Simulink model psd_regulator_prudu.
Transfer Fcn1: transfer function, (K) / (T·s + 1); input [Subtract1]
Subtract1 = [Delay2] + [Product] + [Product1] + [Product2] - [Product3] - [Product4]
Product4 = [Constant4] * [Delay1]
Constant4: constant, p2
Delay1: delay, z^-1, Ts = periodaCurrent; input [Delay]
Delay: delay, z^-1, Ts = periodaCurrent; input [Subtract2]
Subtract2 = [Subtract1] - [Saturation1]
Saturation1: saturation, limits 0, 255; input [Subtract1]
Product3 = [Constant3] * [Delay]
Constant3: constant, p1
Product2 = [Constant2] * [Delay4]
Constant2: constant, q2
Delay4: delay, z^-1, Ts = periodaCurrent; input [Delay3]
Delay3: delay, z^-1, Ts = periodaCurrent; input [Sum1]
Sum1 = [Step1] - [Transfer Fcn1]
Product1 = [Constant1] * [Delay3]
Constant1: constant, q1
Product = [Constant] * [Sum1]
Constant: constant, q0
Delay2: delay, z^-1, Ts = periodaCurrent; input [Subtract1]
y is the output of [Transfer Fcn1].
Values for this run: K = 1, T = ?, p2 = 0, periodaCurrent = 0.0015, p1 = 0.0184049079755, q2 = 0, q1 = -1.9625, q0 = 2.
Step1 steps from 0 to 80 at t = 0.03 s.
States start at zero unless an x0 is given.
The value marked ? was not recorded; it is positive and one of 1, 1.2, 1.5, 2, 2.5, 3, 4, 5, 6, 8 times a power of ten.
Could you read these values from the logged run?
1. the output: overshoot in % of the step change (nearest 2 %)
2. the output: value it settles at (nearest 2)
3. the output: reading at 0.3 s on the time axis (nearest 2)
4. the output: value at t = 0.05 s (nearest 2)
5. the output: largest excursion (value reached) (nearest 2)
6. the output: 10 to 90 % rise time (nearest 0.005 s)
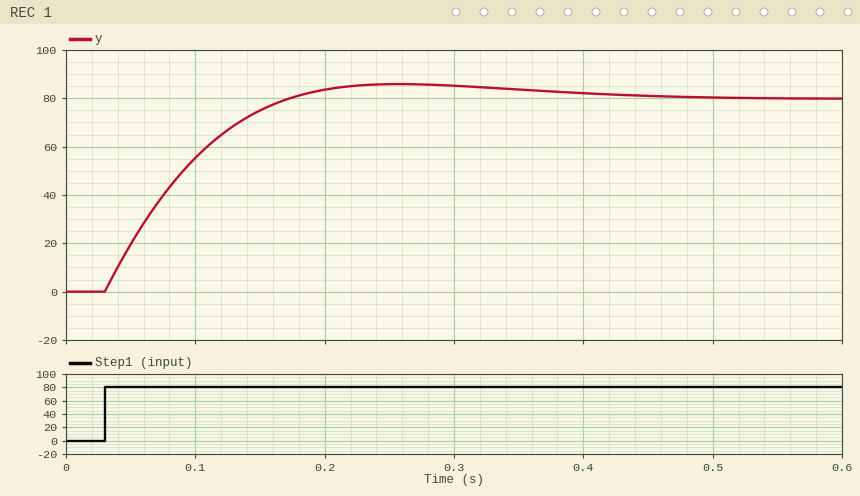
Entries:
8 %
80
86
20
86
0.100 s
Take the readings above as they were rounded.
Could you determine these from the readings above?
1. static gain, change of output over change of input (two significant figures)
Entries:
1.0
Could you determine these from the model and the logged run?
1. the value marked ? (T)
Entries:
0.15
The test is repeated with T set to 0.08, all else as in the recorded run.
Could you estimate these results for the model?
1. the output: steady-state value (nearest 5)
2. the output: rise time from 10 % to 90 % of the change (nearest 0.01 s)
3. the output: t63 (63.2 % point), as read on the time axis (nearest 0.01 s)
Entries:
80
0.09 s
0.07 s
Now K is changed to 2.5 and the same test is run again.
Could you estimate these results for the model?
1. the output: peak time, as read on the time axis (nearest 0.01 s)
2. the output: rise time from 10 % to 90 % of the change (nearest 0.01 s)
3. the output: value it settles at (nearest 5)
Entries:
0.15 s
0.05 s
80
